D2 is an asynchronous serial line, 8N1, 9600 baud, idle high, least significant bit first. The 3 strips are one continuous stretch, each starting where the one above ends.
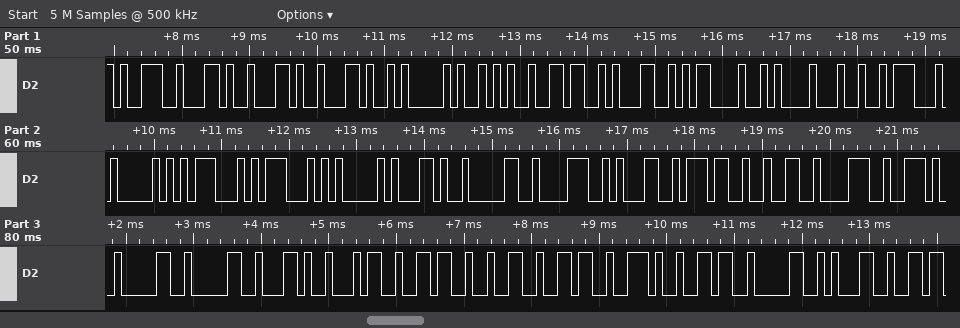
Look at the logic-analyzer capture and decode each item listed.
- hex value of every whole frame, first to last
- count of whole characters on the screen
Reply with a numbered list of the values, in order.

1. 39 2C 2C 2C 41 2A 36 31 0D 0A 24 47 50 47 47 41 2C 30 38 31 37 32 38 2E 30 30 2C 34 36 32 36 2E 36 30 31
2. 35
